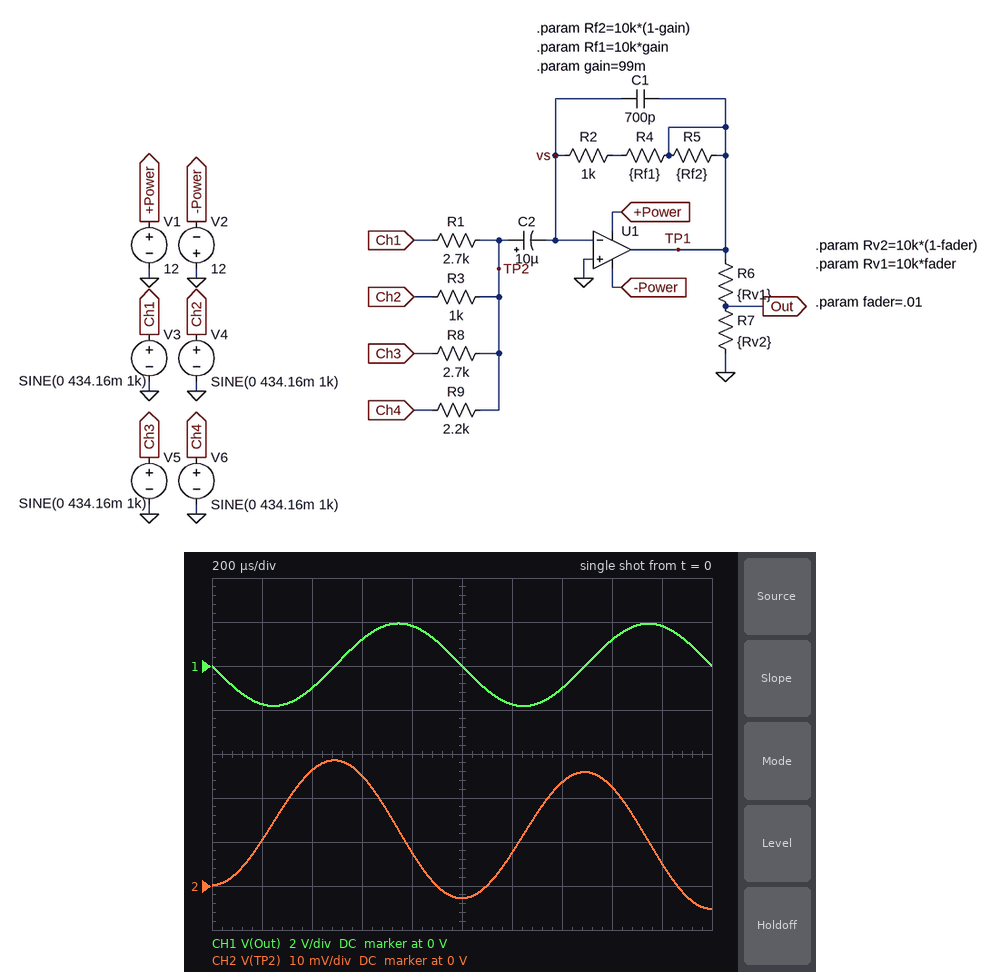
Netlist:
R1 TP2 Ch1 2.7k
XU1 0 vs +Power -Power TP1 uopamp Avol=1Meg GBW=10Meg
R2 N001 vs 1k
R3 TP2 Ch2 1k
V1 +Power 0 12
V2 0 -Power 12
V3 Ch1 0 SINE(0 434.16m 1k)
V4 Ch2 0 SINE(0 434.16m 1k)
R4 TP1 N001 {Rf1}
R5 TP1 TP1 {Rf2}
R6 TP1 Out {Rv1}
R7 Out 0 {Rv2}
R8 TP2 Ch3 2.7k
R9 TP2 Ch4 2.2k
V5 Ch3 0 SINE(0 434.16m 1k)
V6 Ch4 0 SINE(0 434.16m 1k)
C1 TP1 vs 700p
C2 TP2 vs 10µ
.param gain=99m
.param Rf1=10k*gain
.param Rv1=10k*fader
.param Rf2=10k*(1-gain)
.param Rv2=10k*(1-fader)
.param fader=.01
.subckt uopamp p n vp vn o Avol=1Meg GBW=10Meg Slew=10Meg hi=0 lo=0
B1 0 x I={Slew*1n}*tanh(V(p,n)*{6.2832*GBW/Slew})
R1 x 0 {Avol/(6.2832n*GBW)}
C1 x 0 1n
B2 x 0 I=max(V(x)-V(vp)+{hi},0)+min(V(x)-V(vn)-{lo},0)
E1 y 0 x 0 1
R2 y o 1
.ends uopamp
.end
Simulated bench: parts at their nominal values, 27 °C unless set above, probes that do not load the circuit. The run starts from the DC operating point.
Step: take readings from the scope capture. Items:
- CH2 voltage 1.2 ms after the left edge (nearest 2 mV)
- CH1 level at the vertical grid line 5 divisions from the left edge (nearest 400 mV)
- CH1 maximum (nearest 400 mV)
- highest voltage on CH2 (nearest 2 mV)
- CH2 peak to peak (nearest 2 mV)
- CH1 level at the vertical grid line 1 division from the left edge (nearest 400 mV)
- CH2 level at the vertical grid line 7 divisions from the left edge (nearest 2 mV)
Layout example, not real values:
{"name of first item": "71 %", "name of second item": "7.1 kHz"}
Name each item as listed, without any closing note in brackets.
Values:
{"CH2 voltage 1.2 ms after the left edge": "8 mV", "CH1 level at the vertical grid line 5 divisions from the left edge": "0 V", "CH1 maximum": "2.0 V", "highest voltage on CH2": "28 mV", "CH2 peak to peak": "34 mV", "CH1 level at the vertical grid line 1 division from the left edge": "-1.6 V", "CH2 level at the vertical grid line 7 divisions from the left edge": "24 mV"}
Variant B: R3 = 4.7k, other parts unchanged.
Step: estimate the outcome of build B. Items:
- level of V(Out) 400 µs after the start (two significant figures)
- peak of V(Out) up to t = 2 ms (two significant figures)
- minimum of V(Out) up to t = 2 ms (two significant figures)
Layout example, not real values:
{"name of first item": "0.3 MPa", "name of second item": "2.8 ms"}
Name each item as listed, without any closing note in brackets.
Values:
{"level of V(Out) 400 µs after the start": "-670 mV", "peak of V(Out) up to t = 2 ms": "1.2 V", "minimum of V(Out) up to t = 2 ms": "-1.2 V"}
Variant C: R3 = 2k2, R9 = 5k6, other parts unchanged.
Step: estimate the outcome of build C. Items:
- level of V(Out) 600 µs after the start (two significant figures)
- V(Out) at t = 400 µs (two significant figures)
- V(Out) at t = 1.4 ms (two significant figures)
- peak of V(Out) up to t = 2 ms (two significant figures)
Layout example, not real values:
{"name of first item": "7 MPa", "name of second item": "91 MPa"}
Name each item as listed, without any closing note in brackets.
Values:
{"level of V(Out) 600 µs after the start": "730 mV", "V(Out) at t = 400 µs": "-650 mV", "V(Out) at t = 1.4 ms": "-660 mV", "peak of V(Out) up to t = 2 ms": "1.2 V"}
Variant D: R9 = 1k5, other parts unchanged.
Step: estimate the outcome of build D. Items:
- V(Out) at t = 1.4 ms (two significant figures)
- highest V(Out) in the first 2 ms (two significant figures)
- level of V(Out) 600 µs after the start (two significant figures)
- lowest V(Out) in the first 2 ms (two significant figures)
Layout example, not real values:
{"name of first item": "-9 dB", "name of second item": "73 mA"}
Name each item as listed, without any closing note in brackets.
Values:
{"V(Out) at t = 1.4 ms": "-1.1 V", "highest V(Out) in the first 2 ms": "2.1 V", "level of V(Out) 600 µs after the start": "1.3 V", "lowest V(Out) in the first 2 ms": "-2.0 V"}
